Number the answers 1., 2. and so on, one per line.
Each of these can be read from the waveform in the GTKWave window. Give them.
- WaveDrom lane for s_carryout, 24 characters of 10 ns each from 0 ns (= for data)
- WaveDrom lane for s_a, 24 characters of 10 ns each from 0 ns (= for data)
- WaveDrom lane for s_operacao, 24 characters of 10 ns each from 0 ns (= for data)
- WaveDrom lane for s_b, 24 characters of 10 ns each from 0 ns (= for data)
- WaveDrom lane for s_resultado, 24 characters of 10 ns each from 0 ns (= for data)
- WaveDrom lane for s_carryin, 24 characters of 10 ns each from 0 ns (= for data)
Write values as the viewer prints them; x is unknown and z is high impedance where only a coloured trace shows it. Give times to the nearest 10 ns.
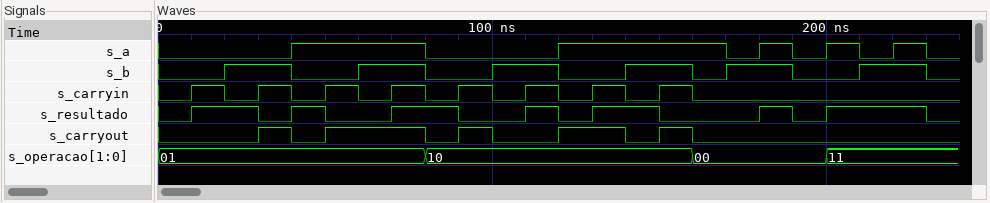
1. {name: 's_carryout', wave: '0..101..010.1.010.......'}
2. {name: 's_a', wave: '0...1...0...1....0101010'}
3. {name: 's_operacao', wave: '=.......=.......=...=...', data: '01 10 00 11'}
4. {name: 's_b', wave: '0.1.0.1.0.1.0.1.01.0.1.0'}
5. {name: 's_resultado', wave: '01.010.1.0.101.0..101..0'}
6. {name: 's_carryin', wave: '01010101010101010.......'}
